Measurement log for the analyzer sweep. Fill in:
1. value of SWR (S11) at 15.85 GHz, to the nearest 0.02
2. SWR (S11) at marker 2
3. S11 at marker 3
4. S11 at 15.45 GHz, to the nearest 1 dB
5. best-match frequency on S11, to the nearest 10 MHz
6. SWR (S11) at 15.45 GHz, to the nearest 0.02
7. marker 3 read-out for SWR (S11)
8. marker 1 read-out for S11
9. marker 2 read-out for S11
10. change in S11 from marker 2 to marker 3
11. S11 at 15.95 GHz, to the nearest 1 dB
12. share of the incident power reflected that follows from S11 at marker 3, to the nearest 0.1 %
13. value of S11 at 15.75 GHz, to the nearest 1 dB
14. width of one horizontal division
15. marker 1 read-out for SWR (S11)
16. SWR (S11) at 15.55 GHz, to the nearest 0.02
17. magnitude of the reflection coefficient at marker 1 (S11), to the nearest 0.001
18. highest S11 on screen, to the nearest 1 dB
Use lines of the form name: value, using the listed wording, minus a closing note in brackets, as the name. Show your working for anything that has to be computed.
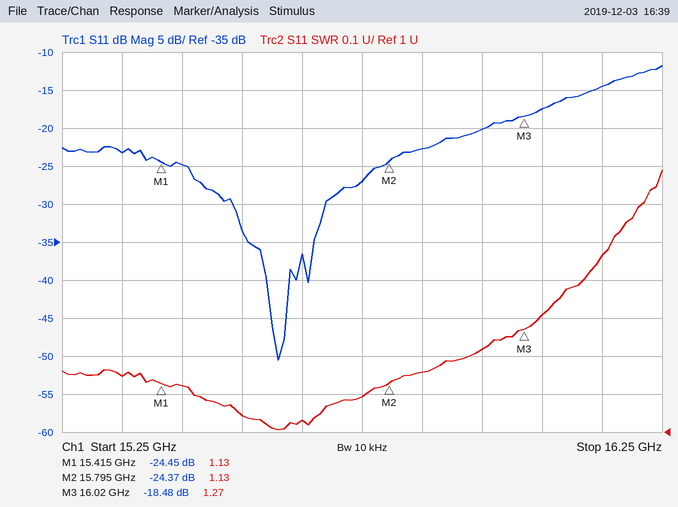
value of SWR (S11) at 15.85 GHz, to the nearest 0.02: 1.16
SWR (S11) at marker 2: 1.13
S11 at marker 3: -18.48 dB
S11 at 15.45 GHz, to the nearest 1 dB: -25 dB
best-match frequency on S11, to the nearest 10 MHz: 15.61 GHz
SWR (S11) at 15.45 GHz, to the nearest 0.02: 1.12
marker 3 read-out for SWR: 1.27
marker 1 read-out for S11: -24.45 dB
marker 2 read-out for S11: -24.37 dB
change in S11 from marker 2 to marker 3: -18.48 − (-24.37) = 5.89 dB
S11 at 15.95 GHz, to the nearest 1 dB: -20 dB
share of the incident power reflected that follows from S11 at marker 3, to the nearest 0.1 %: 10^(-18.48/10) ≈ 1.4 %
value of S11 at 15.75 GHz, to the nearest 1 dB: -27 dB
width of one horizontal division: 100 MHz
marker 1 read-out for SWR: 1.13
SWR (S11) at 15.55 GHz, to the nearest 0.02: 1.04
magnitude of the reflection coefficient at marker 1 (S11), to the nearest 0.001: 10^(-24.45/20) ≈ 0.060
highest S11 on screen, to the nearest 1 dB: -12 dB
